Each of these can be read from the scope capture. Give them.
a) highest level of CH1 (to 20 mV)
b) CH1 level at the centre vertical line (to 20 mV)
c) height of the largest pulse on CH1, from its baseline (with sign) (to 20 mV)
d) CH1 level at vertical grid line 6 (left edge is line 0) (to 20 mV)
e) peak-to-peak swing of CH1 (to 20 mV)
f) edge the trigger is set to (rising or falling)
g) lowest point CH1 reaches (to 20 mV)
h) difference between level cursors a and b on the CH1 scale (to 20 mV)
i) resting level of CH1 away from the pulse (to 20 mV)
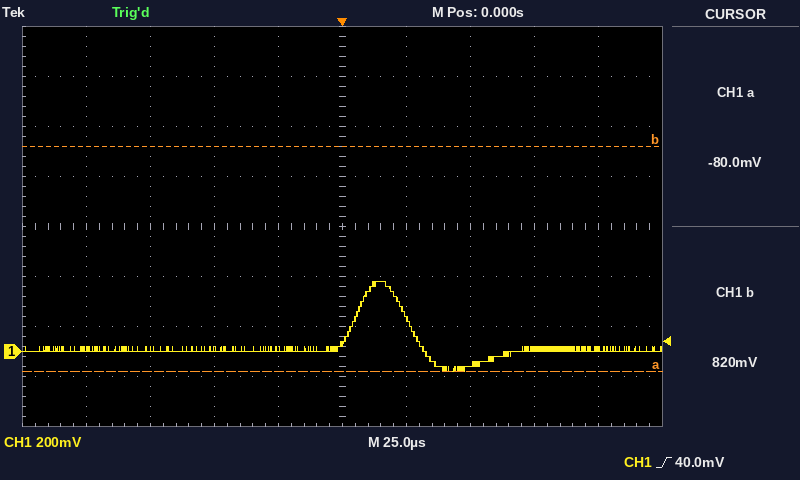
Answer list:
280 mV
40 mV
+280 mV
140 mV
360 mV
rising
-80 mV
900 mV
0 mV
